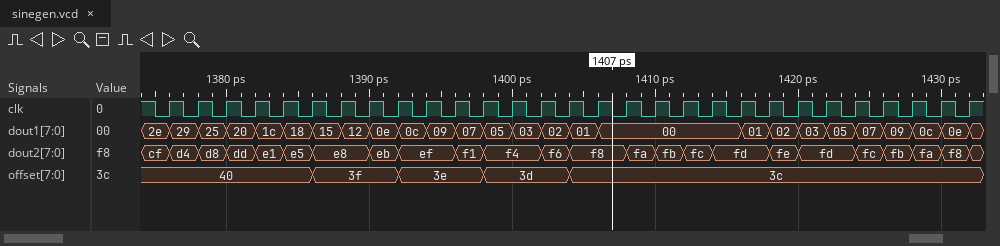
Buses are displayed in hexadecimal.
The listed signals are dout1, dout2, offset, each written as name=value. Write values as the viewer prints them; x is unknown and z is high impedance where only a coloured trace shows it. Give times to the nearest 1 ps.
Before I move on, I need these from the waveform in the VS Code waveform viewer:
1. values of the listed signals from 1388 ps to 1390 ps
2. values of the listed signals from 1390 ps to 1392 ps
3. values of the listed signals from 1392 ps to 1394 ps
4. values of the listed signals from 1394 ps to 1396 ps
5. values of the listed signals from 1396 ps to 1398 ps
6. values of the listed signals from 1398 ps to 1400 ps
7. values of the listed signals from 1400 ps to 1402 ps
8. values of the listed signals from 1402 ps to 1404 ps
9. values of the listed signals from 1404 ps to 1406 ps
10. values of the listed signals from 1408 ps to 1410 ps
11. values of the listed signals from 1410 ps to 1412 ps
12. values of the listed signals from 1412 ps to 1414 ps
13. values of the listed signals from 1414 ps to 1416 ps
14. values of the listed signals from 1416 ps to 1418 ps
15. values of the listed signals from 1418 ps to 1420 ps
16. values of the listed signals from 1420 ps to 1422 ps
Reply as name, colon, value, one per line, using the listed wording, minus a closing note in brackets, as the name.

values of the listed signals from 1388 ps to 1390 ps: dout1=12, dout2=e8, offset=3f
values of the listed signals from 1390 ps to 1392 ps: dout1=0e, dout2=eb, offset=3f
values of the listed signals from 1392 ps to 1394 ps: dout1=0c, dout2=ef, offset=3e
values of the listed signals from 1394 ps to 1396 ps: dout1=09, dout2=ef, offset=3e
values of the listed signals from 1396 ps to 1398 ps: dout1=07, dout2=f1, offset=3e
values of the listed signals from 1398 ps to 1400 ps: dout1=05, dout2=f4, offset=3d
values of the listed signals from 1400 ps to 1402 ps: dout1=03, dout2=f4, offset=3d
values of the listed signals from 1402 ps to 1404 ps: dout1=02, dout2=f6, offset=3d
values of the listed signals from 1404 ps to 1406 ps: dout1=01, dout2=f8, offset=3c
values of the listed signals from 1408 ps to 1410 ps: dout1=00, dout2=fa, offset=3c
values of the listed signals from 1410 ps to 1412 ps: dout1=00, dout2=fb, offset=3c
values of the listed signals from 1412 ps to 1414 ps: dout1=00, dout2=fc, offset=3c
values of the listed signals from 1414 ps to 1416 ps: dout1=00, dout2=fd, offset=3c
values of the listed signals from 1416 ps to 1418 ps: dout1=01, dout2=fd, offset=3c
values of the listed signals from 1418 ps to 1420 ps: dout1=02, dout2=fe, offset=3c
values of the listed signals from 1420 ps to 1422 ps: dout1=03, dout2=fd, offset=3c
